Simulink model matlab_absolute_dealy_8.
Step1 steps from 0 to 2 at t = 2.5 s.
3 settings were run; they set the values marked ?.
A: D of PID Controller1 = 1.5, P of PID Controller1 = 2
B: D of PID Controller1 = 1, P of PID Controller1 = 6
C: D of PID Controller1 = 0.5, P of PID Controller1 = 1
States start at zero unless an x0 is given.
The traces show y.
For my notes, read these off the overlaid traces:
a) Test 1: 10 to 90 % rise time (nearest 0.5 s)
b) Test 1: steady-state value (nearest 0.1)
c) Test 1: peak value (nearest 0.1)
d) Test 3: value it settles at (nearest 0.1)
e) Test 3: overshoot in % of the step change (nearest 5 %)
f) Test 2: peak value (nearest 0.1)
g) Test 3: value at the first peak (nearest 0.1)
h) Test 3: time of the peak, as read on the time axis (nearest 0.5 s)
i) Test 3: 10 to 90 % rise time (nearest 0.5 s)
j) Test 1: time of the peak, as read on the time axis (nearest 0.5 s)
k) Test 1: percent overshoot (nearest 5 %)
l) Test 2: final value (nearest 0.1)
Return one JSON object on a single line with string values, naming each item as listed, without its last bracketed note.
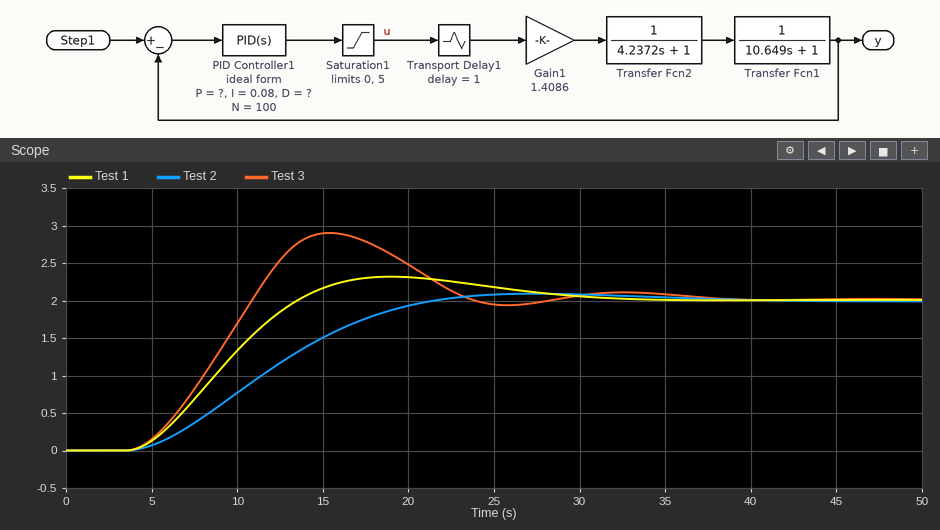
{"Test 1: 10 to 90 % rise time": "7.0 s", "Test 1: steady-state value": "2.0", "Test 1: peak value": "2.3", "Test 3: value it settles at": "2.0", "Test 3: overshoot in % of the step change": "45 %", "Test 2: peak value": "2.1", "Test 3: value at the first peak": "2.9", "Test 3: time of the peak, as read on the time axis": "15.5 s", "Test 3: 10 to 90 % rise time": "5.0 s", "Test 1: time of the peak, as read on the time axis": "19.0 s", "Test 1: percent overshoot": "15 %", "Test 2: final value": "2.0"}
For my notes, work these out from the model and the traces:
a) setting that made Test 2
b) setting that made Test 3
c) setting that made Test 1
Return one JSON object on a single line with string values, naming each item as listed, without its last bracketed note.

{"setting that made Test 2": "C", "setting that made Test 3": "B", "setting that made Test 1": "A"}
